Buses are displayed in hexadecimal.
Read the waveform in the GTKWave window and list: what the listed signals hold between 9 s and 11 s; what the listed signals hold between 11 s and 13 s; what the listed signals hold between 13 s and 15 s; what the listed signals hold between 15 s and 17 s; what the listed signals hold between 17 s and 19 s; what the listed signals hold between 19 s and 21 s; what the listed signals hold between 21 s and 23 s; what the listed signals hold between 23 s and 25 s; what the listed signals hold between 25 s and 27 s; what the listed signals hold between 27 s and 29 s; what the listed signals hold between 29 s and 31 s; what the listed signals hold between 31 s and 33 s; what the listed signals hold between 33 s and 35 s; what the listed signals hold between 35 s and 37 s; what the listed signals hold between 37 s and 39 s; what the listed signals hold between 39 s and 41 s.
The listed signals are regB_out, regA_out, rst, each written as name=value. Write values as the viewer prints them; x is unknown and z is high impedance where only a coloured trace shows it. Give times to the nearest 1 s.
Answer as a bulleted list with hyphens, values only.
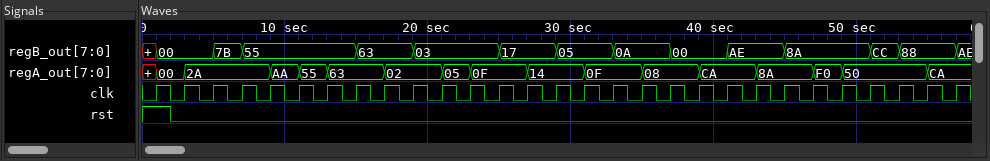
- regB_out=55, regA_out=AA, rst=0
- regB_out=55, regA_out=55, rst=0
- regB_out=55, regA_out=63, rst=0
- regB_out=63, regA_out=63, rst=0
- regB_out=63, regA_out=02, rst=0
- regB_out=03, regA_out=02, rst=0
- regB_out=03, regA_out=05, rst=0
- regB_out=03, regA_out=0F, rst=0
- regB_out=17, regA_out=0F, rst=0
- regB_out=17, regA_out=14, rst=0
- regB_out=05, regA_out=14, rst=0
- regB_out=05, regA_out=0F, rst=0
- regB_out=0A, regA_out=0F, rst=0
- regB_out=0A, regA_out=08, rst=0
- regB_out=00, regA_out=08, rst=0
- regB_out=00, regA_out=CA, rst=0
